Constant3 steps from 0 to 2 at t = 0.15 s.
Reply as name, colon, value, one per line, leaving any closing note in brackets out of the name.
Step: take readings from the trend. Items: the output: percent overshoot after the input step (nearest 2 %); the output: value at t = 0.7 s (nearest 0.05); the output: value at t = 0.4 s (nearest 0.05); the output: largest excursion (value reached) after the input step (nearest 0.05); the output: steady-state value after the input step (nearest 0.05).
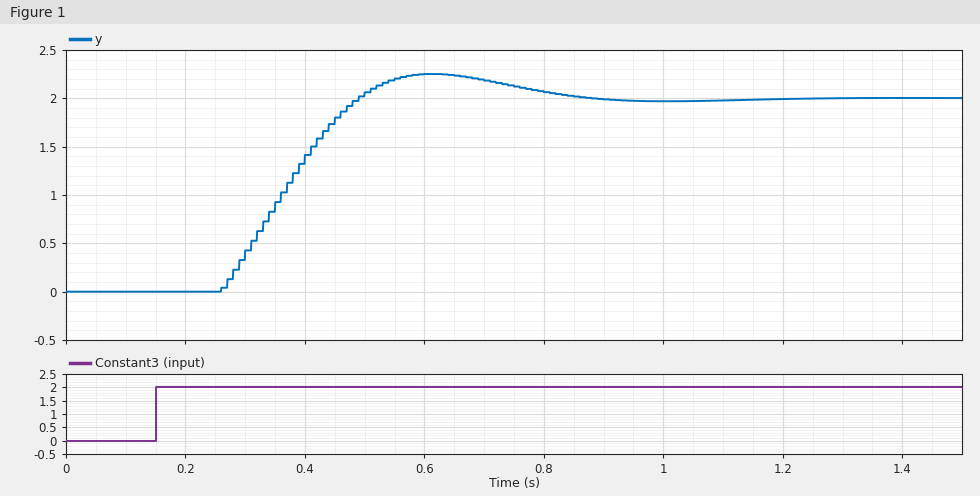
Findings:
the output: percent overshoot after the input step: 12 %
the output: value at t = 0.7 s: 2.20
the output: value at t = 0.4 s: 1.40
the output: largest excursion (value reached) after the input step: 2.25
the output: steady-state value after the input step: 2.00
